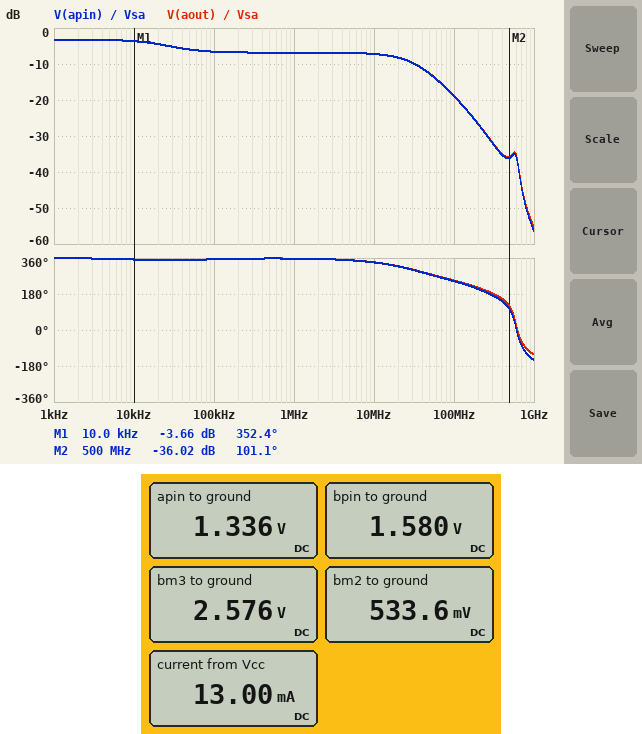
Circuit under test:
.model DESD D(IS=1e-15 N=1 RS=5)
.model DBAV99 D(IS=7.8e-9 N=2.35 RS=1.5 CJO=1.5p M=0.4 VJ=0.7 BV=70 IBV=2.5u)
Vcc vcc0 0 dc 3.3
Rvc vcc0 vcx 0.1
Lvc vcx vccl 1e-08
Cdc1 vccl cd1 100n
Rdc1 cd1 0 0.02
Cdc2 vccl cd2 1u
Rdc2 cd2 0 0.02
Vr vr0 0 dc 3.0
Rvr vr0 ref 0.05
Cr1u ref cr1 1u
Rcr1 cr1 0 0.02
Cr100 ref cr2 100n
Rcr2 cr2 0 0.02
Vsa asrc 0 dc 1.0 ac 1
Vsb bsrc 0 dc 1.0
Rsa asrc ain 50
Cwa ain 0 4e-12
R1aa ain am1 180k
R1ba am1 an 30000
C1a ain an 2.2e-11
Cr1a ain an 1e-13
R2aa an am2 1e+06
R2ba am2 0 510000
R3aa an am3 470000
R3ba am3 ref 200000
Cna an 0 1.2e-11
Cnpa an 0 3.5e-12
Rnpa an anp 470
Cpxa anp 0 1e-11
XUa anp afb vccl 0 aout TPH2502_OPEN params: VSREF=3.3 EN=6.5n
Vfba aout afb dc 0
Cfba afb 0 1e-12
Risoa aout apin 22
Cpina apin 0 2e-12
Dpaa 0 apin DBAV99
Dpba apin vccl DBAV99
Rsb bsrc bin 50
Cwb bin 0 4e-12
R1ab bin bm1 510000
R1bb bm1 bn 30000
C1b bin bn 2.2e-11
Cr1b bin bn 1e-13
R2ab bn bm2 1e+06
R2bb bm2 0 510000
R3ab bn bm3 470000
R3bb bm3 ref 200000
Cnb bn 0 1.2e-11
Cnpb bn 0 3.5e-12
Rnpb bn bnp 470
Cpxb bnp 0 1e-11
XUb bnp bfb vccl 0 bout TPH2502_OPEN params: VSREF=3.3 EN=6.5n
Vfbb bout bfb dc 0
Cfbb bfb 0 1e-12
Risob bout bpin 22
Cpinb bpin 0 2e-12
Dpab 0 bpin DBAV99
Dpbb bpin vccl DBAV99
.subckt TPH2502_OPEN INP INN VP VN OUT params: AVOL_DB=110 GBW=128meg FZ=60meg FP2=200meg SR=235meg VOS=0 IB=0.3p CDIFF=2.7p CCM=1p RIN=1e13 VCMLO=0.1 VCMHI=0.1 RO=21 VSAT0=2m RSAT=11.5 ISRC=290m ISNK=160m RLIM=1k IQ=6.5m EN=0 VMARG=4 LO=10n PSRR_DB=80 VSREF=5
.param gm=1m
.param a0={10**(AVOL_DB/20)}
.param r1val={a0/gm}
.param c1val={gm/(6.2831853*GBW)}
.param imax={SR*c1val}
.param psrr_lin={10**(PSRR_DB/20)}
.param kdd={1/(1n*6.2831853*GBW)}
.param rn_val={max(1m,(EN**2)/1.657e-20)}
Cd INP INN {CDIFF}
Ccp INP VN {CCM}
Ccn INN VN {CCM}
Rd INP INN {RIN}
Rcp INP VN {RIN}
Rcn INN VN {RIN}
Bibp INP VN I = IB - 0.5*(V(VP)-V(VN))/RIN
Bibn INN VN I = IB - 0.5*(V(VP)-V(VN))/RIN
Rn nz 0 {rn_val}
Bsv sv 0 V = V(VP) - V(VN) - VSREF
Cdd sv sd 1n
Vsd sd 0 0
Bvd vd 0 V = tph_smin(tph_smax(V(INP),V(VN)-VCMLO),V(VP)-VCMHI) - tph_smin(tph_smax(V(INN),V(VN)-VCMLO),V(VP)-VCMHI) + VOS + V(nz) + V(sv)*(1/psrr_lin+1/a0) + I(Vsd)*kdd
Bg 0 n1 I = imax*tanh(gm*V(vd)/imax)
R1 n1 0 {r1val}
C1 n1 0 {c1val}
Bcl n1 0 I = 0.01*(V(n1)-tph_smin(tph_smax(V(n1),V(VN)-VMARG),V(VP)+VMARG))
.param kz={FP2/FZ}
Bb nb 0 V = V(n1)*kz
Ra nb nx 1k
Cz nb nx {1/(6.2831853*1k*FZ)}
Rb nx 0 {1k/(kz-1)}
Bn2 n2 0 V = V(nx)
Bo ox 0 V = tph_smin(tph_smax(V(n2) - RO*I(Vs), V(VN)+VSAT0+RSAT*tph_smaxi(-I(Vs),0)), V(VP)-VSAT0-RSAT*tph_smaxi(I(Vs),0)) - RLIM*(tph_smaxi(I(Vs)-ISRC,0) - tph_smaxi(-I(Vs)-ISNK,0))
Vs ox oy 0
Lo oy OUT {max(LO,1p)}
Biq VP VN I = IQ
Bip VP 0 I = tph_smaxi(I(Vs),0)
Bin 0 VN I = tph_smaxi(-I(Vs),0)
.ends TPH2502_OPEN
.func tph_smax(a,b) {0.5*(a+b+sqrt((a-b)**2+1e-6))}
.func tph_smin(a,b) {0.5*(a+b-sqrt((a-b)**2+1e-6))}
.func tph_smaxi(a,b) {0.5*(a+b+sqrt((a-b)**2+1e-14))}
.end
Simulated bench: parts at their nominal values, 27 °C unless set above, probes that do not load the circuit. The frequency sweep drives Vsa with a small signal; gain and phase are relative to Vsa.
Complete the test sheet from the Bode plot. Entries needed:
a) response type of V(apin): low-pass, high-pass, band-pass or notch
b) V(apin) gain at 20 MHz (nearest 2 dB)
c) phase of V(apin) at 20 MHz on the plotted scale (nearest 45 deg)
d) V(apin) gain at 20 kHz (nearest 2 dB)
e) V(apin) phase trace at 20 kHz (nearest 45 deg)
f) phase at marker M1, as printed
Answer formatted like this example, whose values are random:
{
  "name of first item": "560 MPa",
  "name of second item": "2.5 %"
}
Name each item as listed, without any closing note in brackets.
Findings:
{
  "response type of V(apin): low-pass, high-pass, band-pass or notch": "low-pass",
  "V(apin) gain at 20 MHz": "-8 dB",
  "phase of V(apin) at 20 MHz on the plotted scale": "315 deg",
  "V(apin) gain at 20 kHz": "-4 dB",
  "V(apin) phase trace at 20 kHz": "360 deg",
  "phase at marker M1, as printed": "352.4 deg"
}
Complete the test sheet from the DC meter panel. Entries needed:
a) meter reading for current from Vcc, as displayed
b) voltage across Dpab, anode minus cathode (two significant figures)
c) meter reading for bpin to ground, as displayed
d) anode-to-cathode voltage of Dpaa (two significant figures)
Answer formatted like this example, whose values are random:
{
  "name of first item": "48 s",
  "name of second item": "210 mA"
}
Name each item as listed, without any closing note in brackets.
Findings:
{
  "meter reading for current from Vcc, as displayed": "13.00 mA",
  "voltage across Dpab, anode minus cathode": "-1.6 V",
  "meter reading for bpin to ground, as displayed": "1.580 V",
  "anode-to-cathode voltage of Dpaa": "-1.3 V"
}
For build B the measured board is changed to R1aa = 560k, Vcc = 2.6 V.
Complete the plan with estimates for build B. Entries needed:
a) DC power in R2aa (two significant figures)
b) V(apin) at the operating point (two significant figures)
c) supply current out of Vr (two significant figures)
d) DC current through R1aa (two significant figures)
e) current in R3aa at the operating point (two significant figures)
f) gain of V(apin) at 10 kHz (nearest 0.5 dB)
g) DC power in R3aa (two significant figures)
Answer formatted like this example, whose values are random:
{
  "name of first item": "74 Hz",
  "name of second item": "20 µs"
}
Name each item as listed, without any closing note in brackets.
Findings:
{
  "DC power in R2aa": "1.1 µW",
  "V(apin) at the operating point": "1.6 V",
  "supply current out of Vr": "4.2 µA",
  "DC current through R1aa": "1.0 µA",
  "current in R3aa at the operating point": "2.1 µA",
  "gain of V(apin) at 10 kHz": "-7.0 dB",
  "DC power in R3aa": "2.0 µW"
}
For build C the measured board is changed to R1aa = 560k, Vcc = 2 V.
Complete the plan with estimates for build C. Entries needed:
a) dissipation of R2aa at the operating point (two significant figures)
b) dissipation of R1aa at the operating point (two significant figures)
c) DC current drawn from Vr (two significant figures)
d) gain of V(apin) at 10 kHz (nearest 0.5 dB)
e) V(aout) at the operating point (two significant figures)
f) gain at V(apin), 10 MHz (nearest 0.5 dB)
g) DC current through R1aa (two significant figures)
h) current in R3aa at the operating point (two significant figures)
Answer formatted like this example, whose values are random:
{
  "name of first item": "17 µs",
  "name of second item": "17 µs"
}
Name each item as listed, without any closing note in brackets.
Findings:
{
  "dissipation of R2aa at the operating point": "1.1 µW",
  "dissipation of R1aa at the operating point": "590 nW",
  "DC current drawn from Vr": "4.2 µA",
  "gain of V(apin) at 10 kHz": "-7.0 dB",
  "V(aout) at the operating point": "1.6 V",
  "gain at V(apin), 10 MHz": "-7.0 dB",
  "DC current through R1aa": "1.0 µA",
  "current in R3aa at the operating point": "2.1 µA"
}
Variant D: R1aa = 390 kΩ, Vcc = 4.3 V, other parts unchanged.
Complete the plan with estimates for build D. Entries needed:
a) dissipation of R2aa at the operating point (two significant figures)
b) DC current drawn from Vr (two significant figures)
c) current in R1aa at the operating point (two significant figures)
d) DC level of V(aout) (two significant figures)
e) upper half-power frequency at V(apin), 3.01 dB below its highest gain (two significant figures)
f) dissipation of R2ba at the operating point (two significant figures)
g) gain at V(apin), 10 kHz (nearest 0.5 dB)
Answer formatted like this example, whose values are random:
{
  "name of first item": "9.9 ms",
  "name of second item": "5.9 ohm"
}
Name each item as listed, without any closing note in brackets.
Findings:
{
  "dissipation of R2aa at the operating point": "1.0 µW",
  "DC current drawn from Vr": "4.3 µA",
  "current in R1aa at the operating point": "1.2 µA",
  "DC level of V(aout)": "1.5 V",
  "upper half-power frequency at V(apin), 3.01 dB below its highest gain": "23 MHz",
  "dissipation of R2ba at the operating point": "510 nW",
  "gain at V(apin), 10 kHz": "-6.0 dB"
}
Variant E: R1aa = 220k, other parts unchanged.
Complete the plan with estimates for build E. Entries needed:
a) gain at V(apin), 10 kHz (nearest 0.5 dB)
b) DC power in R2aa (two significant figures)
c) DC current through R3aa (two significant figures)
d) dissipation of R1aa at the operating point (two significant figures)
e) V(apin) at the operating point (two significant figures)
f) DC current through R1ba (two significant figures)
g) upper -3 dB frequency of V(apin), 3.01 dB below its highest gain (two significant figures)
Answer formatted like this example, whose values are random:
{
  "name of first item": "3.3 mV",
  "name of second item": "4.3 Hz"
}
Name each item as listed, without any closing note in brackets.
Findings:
{
  "gain at V(apin), 10 kHz": "-4.0 dB",
  "DC power in R2aa": "830 nW",
  "DC current through R3aa": "2.4 µA",
  "dissipation of R1aa at the operating point": "500 nW",
  "V(apin) at the operating point": "1.4 V",
  "DC current through R1ba": "1.5 µA",
  "upper -3 dB frequency of V(apin), 3.01 dB below its highest gain": "140 kHz"
}
